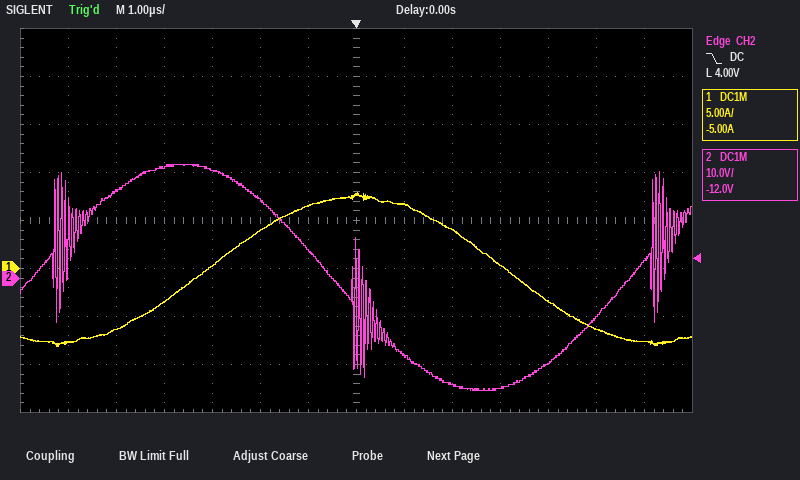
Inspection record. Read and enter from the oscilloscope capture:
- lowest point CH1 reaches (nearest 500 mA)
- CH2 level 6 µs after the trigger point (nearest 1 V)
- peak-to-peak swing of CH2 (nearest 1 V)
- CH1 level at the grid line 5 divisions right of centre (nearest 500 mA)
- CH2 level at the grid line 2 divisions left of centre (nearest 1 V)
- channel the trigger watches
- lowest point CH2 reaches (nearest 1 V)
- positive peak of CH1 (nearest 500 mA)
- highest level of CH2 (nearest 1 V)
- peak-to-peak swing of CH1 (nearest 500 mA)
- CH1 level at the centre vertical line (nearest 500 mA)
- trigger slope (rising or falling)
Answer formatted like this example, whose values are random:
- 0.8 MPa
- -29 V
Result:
- -8.0 A
- 4 V
- 47 V
- -6.5 A
- 16 V
- CH2
- -23 V
- 8.0 A
- 24 V
- 16.0 A
- 7.5 A
- falling
